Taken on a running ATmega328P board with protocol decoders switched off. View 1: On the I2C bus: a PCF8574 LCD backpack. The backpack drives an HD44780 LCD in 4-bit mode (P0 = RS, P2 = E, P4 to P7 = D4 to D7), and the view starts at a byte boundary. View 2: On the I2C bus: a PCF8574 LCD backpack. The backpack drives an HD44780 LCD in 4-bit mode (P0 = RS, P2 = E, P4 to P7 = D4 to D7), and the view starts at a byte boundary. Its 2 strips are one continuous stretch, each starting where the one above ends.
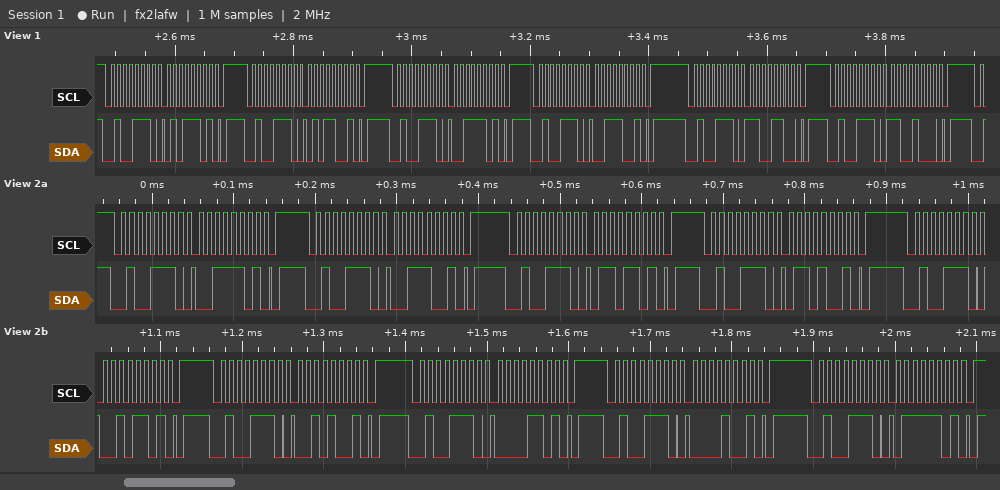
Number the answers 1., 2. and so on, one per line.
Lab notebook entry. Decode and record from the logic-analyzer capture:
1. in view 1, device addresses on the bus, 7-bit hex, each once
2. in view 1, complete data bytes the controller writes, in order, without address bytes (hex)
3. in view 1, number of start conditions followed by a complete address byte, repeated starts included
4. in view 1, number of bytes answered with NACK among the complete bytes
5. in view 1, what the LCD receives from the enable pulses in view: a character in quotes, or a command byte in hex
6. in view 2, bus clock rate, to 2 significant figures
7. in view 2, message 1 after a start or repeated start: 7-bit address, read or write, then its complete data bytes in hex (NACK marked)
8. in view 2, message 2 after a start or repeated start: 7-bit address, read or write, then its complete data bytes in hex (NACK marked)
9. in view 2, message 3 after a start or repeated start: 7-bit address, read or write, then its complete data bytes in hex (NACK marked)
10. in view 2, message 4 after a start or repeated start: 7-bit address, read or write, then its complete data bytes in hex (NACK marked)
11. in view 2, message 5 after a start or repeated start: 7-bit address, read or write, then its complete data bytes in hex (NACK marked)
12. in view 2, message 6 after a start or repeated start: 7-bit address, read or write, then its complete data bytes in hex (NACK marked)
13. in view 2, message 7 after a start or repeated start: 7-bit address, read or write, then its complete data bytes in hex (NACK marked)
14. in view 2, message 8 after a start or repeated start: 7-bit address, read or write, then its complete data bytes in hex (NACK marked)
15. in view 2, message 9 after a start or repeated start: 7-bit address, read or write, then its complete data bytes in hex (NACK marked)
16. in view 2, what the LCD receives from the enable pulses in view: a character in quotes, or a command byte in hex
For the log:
1. 0x27
2. 5D 59 3D 39 CC C8
3. 6
4. 0
5. 'S'
6. 100 kHz
7. 0x27 write: 3D
8. 0x27 write: 39
9. 0x27 write: 6D
10. 0x27 write: 69
11. 0x27 write: 2D
12. 0x27 write: 29
13. 0x27 write: 0D
14. 0x27 write: 09
15. 0x27 write: 7D
16. '6' ' '
